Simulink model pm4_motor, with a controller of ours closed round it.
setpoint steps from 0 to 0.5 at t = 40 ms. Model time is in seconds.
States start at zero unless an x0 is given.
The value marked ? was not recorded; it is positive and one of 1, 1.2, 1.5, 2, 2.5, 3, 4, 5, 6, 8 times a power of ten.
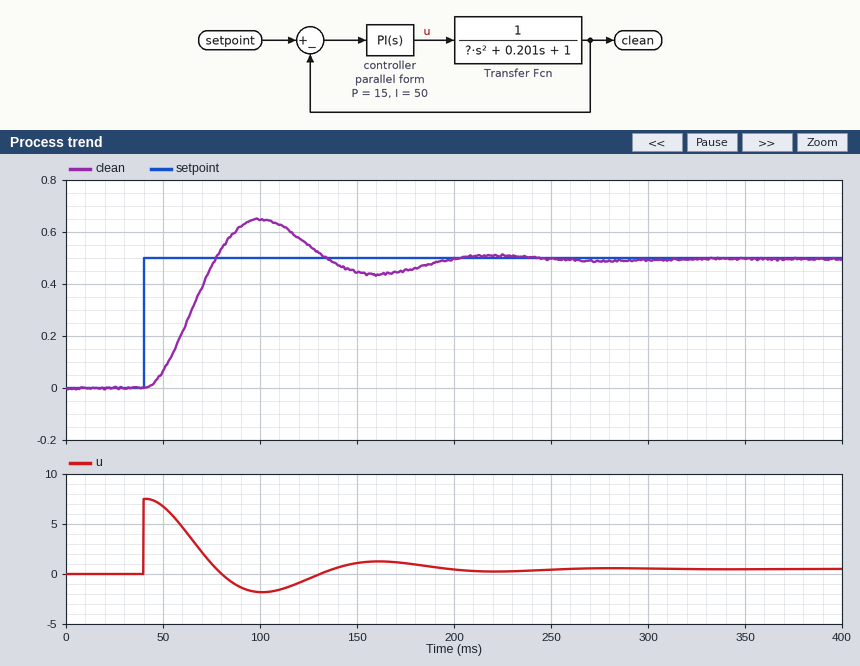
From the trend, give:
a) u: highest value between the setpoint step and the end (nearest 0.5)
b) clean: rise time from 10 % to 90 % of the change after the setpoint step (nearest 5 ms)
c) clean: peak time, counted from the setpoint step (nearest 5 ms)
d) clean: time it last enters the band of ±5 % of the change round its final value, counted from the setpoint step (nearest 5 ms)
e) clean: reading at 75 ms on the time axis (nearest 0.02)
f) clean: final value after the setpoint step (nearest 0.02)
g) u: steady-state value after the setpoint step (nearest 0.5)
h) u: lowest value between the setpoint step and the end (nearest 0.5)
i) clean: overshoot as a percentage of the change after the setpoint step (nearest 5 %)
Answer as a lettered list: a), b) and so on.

a) 7.5
b) 25 ms
c) 60 ms
d) 145 ms
e) 0.46
f) 0.50
g) 0.5
h) -2.0
i) 30 %
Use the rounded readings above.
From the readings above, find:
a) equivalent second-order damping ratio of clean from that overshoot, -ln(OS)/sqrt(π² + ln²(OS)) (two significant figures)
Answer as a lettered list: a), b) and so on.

a) 0.36
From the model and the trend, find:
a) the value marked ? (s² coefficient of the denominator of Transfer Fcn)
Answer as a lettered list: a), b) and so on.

a) 0.005
